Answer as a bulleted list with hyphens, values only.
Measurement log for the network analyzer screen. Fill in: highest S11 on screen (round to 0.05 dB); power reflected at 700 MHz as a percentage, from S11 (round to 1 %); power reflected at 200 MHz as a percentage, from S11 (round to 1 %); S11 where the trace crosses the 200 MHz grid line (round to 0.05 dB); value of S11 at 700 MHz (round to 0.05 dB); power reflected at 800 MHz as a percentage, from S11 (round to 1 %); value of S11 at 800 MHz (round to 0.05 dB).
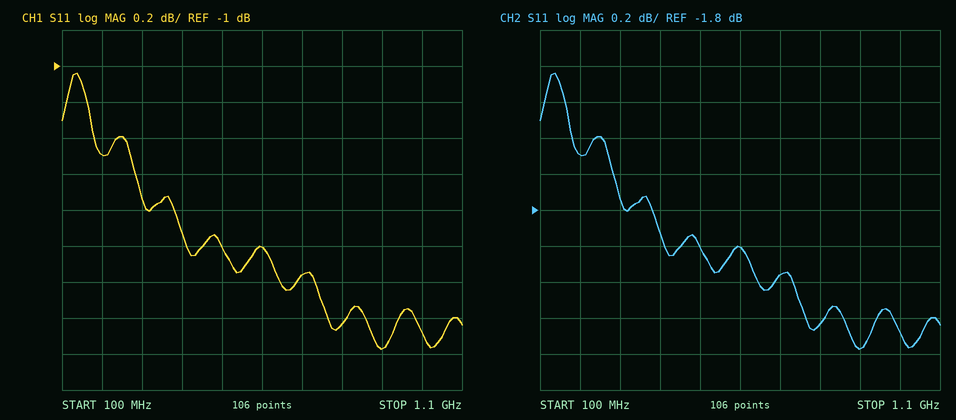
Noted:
- -1.05 dB
- 61 %
- 71 %
- -1.50 dB
- -2.15 dB
- 57 %
- -2.45 dB
